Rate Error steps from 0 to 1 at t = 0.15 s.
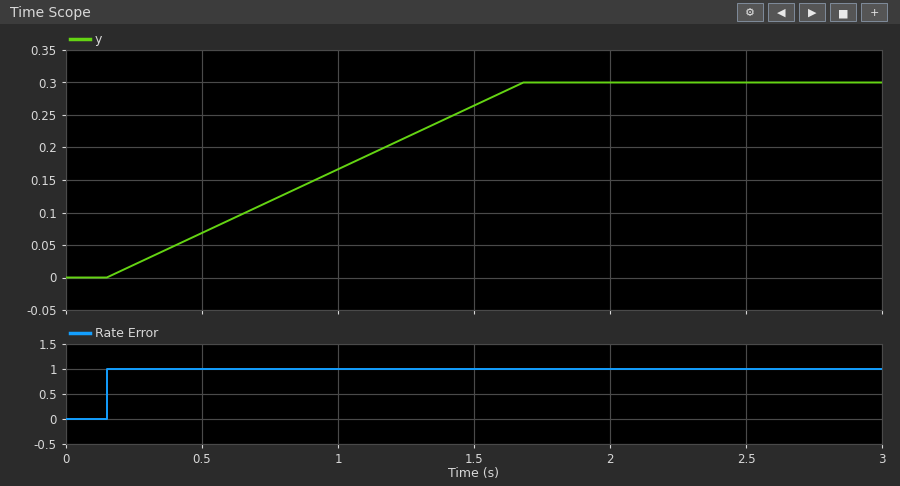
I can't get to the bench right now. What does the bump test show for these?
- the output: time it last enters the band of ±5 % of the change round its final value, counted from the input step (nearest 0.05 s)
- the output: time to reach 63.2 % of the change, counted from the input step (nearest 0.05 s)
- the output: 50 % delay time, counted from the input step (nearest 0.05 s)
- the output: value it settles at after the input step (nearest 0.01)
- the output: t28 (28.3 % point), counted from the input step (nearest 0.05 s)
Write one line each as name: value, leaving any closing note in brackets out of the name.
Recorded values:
the output: time it last enters the band of ±5 % of the change round its final value, counted from the input step: 1.45 s
the output: time to reach 63.2 % of the change, counted from the input step: 0.95 s
the output: 50 % delay time, counted from the input step: 0.75 s
the output: value it settles at after the input step: 0.30
the output: t28 (28.3 % point), counted from the input step: 0.45 s
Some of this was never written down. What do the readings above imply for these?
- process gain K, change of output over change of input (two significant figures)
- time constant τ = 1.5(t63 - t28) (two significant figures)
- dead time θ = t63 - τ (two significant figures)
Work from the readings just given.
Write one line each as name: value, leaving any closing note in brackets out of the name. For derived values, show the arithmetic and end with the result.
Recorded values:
process gain K, change of output over change of input: (0.3 - 0) / 1 = 0.30
time constant τ = 1.5(t63 - t28): 1.5 × (0.95 - 0.45) = 0.75 s
dead time θ = t63 - τ: 0.95 - 0.75 = 0.20 s
